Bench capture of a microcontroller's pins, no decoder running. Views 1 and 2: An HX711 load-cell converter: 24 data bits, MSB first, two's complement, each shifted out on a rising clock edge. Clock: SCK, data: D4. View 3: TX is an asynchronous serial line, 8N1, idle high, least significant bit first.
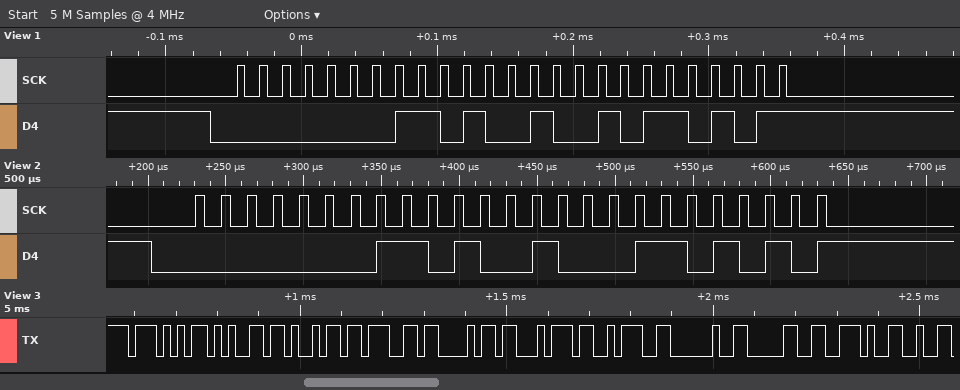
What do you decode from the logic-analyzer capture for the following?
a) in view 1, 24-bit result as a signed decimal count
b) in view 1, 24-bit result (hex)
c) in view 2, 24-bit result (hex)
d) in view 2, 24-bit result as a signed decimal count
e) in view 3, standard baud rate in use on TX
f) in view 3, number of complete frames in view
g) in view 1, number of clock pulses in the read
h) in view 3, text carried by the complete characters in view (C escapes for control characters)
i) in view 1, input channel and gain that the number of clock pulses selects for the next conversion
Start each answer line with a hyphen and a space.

- 107701
- 0x01A4B5
- 0x01A46A
- 107626
- 57600 baud
- 10
- 25
- "Weight: 0."
- channel A, gain 128
